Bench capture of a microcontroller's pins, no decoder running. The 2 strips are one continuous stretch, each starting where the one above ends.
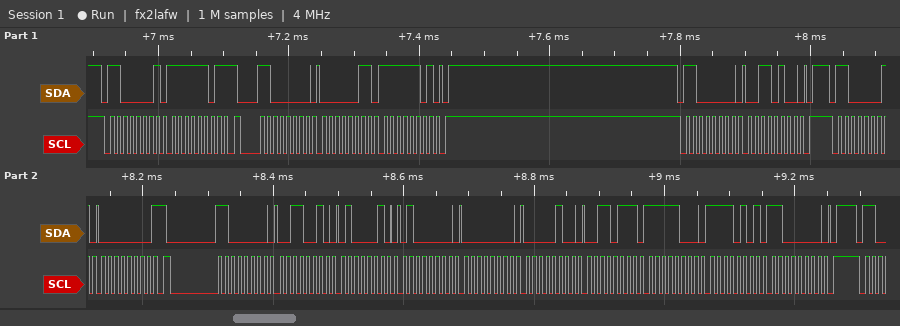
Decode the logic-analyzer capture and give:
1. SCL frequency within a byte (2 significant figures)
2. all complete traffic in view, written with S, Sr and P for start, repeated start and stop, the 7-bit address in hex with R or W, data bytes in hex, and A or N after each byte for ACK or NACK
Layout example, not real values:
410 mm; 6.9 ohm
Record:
100 kHz; S 60R A FD N Sr 60W A 03 A FD A P S 60W A 34 A P S 60R A 00 N Sr 60W A 32 A 42 A 40 A 00 A 04 A 37 A F8 A F5 A C0 A P
